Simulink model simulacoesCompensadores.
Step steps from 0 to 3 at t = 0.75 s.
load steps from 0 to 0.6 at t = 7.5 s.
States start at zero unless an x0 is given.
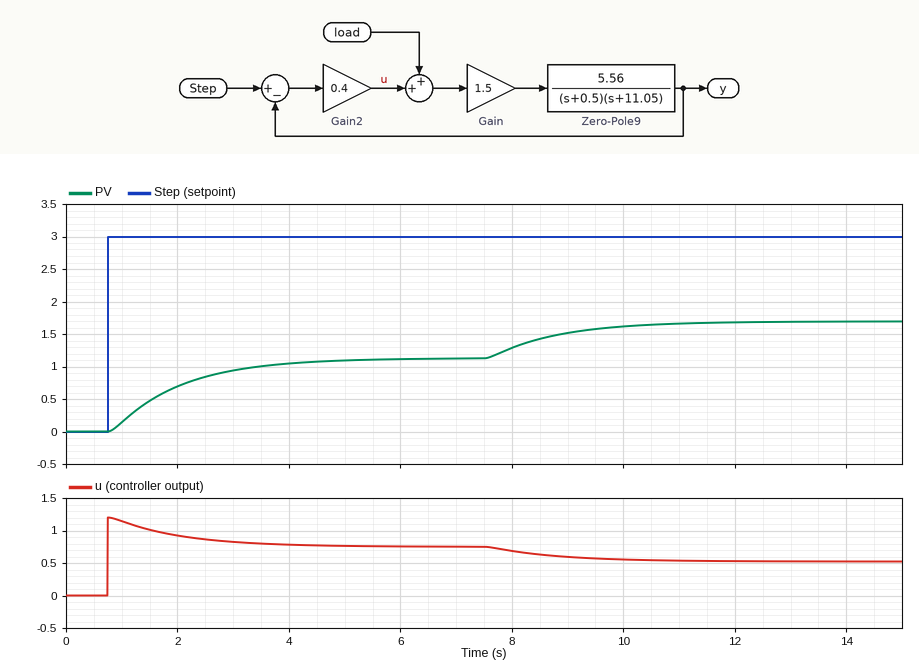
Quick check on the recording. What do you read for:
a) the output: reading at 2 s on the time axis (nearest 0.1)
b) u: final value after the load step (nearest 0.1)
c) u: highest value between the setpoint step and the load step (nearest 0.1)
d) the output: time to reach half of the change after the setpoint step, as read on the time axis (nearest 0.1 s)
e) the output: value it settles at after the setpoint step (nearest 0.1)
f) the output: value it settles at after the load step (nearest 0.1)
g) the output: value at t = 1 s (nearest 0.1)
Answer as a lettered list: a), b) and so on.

a) 0.7
b) 0.5
c) 1.2
d) 1.7 s
e) 1.1
f) 1.7
g) 0.1
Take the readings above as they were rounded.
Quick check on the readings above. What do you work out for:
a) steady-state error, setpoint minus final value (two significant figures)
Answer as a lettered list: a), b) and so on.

a) 1.9
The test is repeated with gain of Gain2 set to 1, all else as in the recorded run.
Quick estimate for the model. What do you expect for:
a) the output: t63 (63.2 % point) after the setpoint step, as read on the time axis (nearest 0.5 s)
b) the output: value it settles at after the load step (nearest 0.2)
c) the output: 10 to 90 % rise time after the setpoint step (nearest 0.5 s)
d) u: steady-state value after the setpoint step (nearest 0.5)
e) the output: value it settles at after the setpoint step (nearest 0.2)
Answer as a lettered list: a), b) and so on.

a) 1.5 s
b) 2.2
c) 1.5 s
d) 1.0
e) 1.8
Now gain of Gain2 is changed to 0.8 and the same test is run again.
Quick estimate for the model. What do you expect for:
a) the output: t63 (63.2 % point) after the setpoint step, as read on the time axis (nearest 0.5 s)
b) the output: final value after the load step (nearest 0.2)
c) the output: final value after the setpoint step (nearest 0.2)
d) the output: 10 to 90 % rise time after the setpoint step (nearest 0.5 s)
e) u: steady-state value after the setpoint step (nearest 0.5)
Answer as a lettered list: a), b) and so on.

a) 1.5 s
b) 2.0
c) 1.6
d) 2.0 s
e) 1.0
